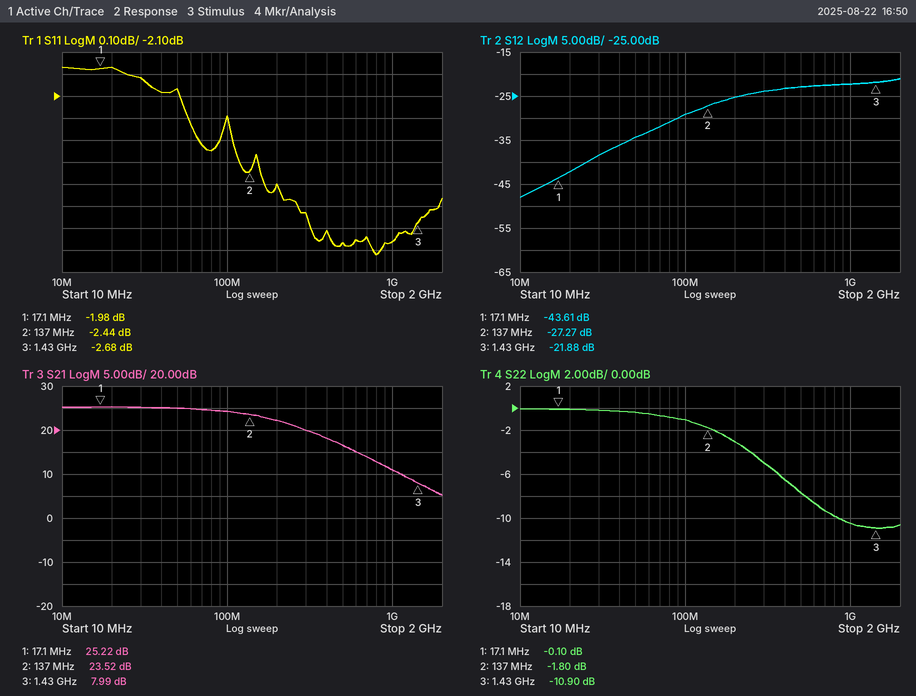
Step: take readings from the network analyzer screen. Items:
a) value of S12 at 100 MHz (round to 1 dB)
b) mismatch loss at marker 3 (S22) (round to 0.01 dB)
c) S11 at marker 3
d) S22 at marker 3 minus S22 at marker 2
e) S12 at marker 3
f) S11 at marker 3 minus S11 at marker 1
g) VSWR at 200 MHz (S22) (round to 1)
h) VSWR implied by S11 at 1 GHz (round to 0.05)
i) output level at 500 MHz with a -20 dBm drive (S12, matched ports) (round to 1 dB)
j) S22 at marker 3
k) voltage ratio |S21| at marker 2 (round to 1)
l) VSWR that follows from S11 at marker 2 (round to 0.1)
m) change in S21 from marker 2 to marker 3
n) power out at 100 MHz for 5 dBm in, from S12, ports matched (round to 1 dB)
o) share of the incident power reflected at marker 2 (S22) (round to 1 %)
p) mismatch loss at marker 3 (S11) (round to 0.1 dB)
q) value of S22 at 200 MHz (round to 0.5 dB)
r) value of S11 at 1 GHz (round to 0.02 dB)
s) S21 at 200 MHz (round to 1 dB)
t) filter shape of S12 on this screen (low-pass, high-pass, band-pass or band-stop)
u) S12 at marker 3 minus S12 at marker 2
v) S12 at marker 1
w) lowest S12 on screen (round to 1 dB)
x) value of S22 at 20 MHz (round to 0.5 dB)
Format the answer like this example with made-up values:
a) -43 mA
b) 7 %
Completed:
a) -29 dB
b) 0.37 dB
c) -2.68 dB
d) -9.10 dB
e) -21.88 dB
f) -0.70 dB
g) 6
h) 6.35
i) -43 dBm
j) -10.90 dB
k) 15
l) 7.2
m) -15.53 dB
n) -24 dBm
o) 66 %
p) 3.4 dB
q) -3.0 dB
r) -2.76 dB
s) 22 dB
t) high-pass
u) 5.39 dB
v) -43.61 dB
w) -48 dB
x) 0.0 dB
